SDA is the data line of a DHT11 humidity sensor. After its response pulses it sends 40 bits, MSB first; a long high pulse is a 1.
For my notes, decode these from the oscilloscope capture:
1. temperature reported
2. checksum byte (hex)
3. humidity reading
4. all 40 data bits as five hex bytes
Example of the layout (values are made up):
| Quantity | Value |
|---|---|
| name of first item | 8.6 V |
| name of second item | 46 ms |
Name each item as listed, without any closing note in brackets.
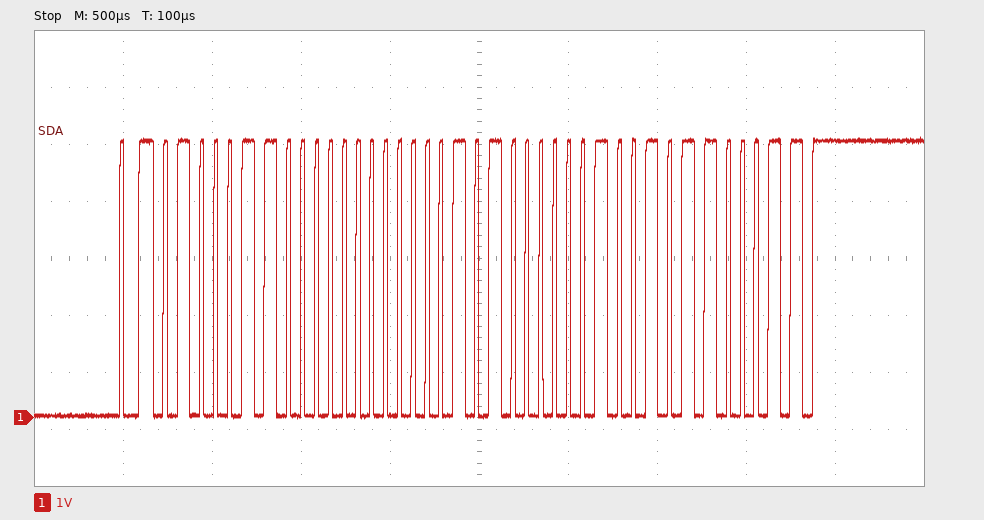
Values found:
| Quantity | Value |
|---|---|
| temperature reported | 20.9 °C |
| checksum byte | 0x63 |
| humidity reading | 70 % |
| all 40 data bits as five hex bytes | 46 00 14 09 63 |
